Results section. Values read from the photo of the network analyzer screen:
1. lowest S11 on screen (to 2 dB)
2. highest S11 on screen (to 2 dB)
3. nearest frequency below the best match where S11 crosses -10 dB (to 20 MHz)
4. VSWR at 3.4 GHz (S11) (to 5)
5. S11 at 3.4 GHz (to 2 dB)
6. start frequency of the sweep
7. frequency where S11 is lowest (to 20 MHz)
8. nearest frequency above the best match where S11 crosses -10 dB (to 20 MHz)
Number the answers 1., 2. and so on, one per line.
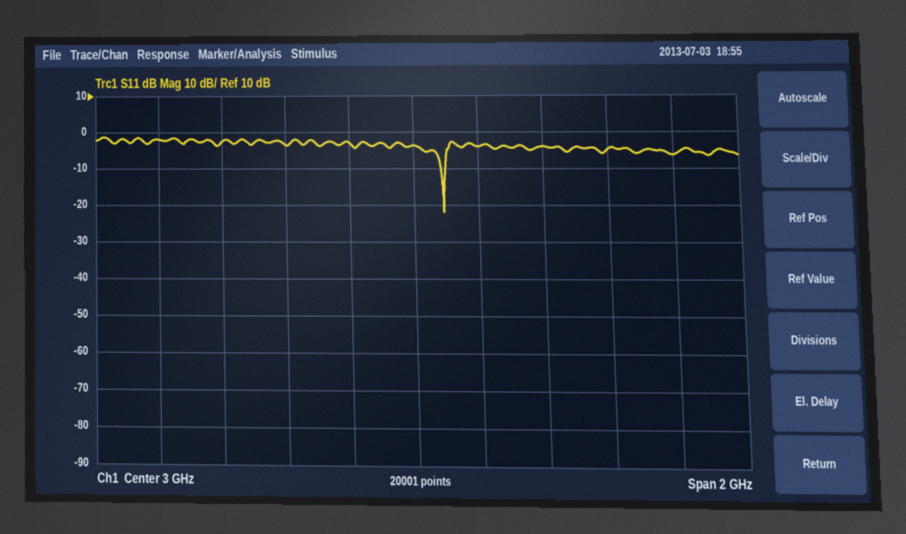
1. -22 dB
2. -2 dB
3. 3.08 GHz
4. 5
5. -4 dB
6. 2 GHz
7. 3.10 GHz
8. 3.10 GHz
